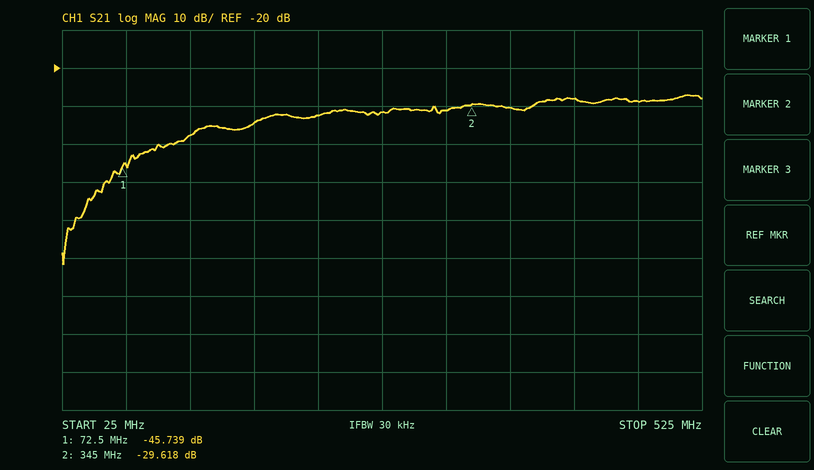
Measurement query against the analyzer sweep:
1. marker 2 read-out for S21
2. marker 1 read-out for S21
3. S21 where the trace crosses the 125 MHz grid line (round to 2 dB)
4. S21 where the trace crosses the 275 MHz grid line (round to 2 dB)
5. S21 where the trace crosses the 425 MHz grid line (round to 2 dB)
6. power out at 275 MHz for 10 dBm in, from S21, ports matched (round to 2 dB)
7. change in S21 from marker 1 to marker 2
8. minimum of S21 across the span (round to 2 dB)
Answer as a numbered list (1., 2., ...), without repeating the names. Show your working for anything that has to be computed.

1. -29.618 dB
2. -45.739 dB
3. -38 dB
4. -32 dB
5. -28 dB
6. 10 dBm + (-32 dB) = -22 dBm
7. -29.618 − (-45.739) = 16.121 dB
8. -72 dB
